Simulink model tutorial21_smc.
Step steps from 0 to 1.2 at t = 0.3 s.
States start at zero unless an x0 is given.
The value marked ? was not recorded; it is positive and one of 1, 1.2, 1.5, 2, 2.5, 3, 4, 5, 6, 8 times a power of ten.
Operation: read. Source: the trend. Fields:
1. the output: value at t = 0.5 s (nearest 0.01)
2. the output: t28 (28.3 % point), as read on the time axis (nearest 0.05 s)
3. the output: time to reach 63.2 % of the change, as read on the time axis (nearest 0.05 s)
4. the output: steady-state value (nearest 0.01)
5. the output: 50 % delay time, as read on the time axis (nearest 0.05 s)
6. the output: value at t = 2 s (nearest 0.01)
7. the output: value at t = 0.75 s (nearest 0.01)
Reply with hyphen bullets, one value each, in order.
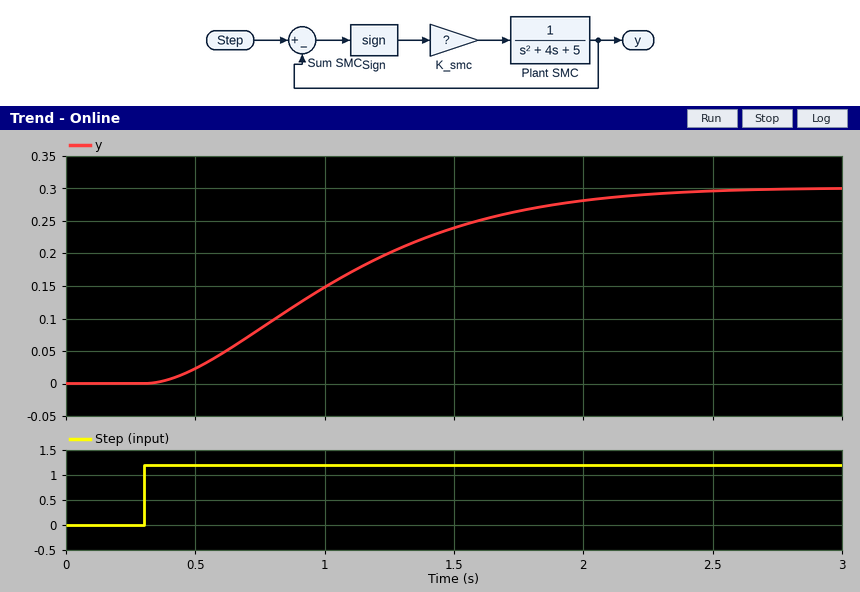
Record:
- 0.02
- 0.75 s
- 1.20 s
- 0.30
- 1.00 s
- 0.28
- 0.08
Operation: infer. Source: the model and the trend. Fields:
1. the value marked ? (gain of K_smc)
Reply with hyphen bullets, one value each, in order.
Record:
- 1.5
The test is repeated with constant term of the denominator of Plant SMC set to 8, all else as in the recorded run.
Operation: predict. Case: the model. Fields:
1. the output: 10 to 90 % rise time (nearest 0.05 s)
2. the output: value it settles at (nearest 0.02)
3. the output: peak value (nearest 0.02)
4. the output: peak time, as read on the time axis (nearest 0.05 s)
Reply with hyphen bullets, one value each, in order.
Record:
- 0.75 s
- 0.18
- 0.20
- 1.85 s
